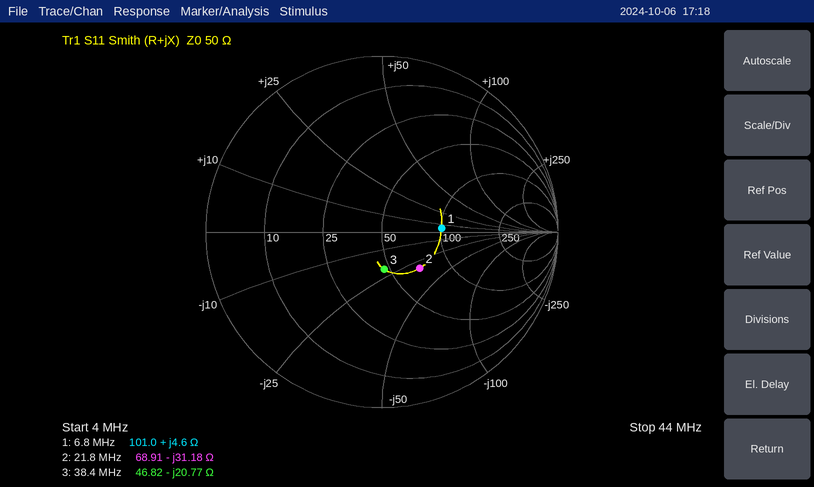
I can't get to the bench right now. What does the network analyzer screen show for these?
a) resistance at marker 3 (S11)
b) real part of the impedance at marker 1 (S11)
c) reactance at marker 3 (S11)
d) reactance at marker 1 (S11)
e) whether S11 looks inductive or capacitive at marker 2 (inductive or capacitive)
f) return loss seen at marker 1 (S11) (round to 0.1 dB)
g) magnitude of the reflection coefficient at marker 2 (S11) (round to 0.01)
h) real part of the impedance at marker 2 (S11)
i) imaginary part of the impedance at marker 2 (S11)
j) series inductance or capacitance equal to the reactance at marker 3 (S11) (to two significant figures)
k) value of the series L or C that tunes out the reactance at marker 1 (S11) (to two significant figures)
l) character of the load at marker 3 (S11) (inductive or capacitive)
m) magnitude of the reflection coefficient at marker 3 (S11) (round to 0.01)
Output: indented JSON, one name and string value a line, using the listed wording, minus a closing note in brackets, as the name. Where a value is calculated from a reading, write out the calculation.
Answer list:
{
  "resistance at marker 3": "46.82 Ω",
  "real part of the impedance at marker 1": "101.0 Ω",
  "reactance at marker 3": "-20.77 Ω",
  "reactance at marker 1": "+4.6 Ω",
  "whether S11 looks inductive or capacitive at marker 2": "capacitive",
  "return loss seen at marker 1 (S11)": "9.4 dB",
  "magnitude of the reflection coefficient at marker 2 (S11)": "0.30",
  "real part of the impedance at marker 2": "68.91 Ω",
  "imaginary part of the impedance at marker 2": "-31.18 Ω",
  "series inductance or capacitance equal to the reactance at marker 3 (S11)": "C = 1/(2π × 38.4 MHz × 20.77 Ω) ≈ 200 pF",
  "value of the series L or C that tunes out the reactance at marker 1 (S11)": "C = 1/(2π × 6.8 MHz × 4.6 Ω) ≈ 5.1 nF",
  "character of the load at marker 3 (S11)": "capacitive",
  "magnitude of the reflection coefficient at marker 3 (S11)": "0.21"
}
